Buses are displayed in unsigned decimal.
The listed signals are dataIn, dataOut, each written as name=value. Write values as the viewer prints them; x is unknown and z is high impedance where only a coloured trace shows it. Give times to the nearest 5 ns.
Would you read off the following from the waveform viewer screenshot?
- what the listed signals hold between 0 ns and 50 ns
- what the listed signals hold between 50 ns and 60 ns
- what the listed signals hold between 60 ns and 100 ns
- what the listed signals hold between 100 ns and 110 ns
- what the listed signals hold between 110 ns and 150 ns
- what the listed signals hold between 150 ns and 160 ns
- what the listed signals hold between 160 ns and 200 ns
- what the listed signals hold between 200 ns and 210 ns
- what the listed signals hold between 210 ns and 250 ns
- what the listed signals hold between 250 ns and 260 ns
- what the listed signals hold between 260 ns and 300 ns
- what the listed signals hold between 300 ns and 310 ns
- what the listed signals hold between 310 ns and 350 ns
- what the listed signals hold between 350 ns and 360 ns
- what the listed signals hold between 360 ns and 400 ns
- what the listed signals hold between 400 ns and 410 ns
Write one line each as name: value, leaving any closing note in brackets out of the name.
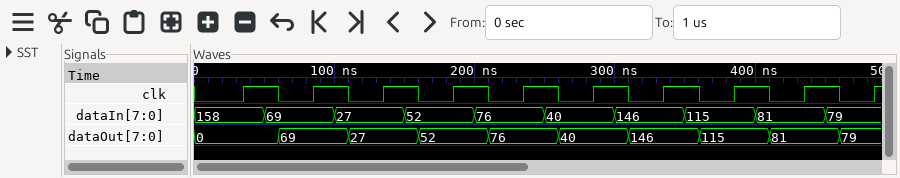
what the listed signals hold between 0 ns and 50 ns: dataIn=158, dataOut=0
what the listed signals hold between 50 ns and 60 ns: dataIn=69, dataOut=0
what the listed signals hold between 60 ns and 100 ns: dataIn=69, dataOut=69
what the listed signals hold between 100 ns and 110 ns: dataIn=27, dataOut=69
what the listed signals hold between 110 ns and 150 ns: dataIn=27, dataOut=27
what the listed signals hold between 150 ns and 160 ns: dataIn=52, dataOut=27
what the listed signals hold between 160 ns and 200 ns: dataIn=52, dataOut=52
what the listed signals hold between 200 ns and 210 ns: dataIn=76, dataOut=52
what the listed signals hold between 210 ns and 250 ns: dataIn=76, dataOut=76
what the listed signals hold between 250 ns and 260 ns: dataIn=40, dataOut=76
what the listed signals hold between 260 ns and 300 ns: dataIn=40, dataOut=40
what the listed signals hold between 300 ns and 310 ns: dataIn=146, dataOut=40
what the listed signals hold between 310 ns and 350 ns: dataIn=146, dataOut=146
what the listed signals hold between 350 ns and 360 ns: dataIn=115, dataOut=146
what the listed signals hold between 360 ns and 400 ns: dataIn=115, dataOut=115
what the listed signals hold between 400 ns and 410 ns: dataIn=81, dataOut=115
